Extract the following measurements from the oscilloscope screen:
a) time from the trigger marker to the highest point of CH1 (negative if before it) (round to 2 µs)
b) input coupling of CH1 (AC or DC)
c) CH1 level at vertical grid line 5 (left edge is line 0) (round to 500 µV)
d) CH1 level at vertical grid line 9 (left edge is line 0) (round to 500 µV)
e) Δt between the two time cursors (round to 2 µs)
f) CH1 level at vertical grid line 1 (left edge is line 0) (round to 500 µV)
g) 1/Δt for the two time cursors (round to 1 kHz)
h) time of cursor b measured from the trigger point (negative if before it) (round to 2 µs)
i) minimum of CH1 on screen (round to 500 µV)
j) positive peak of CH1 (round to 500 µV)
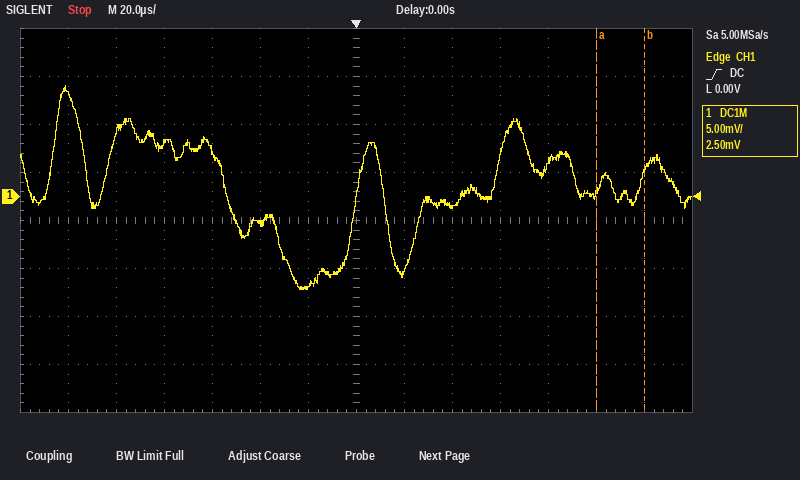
-122 µs
DC
-3.0 mV
-1.0 mV
20 µs
10.5 mV
50 kHz
+120 µs
-9.5 mV
11.5 mV
